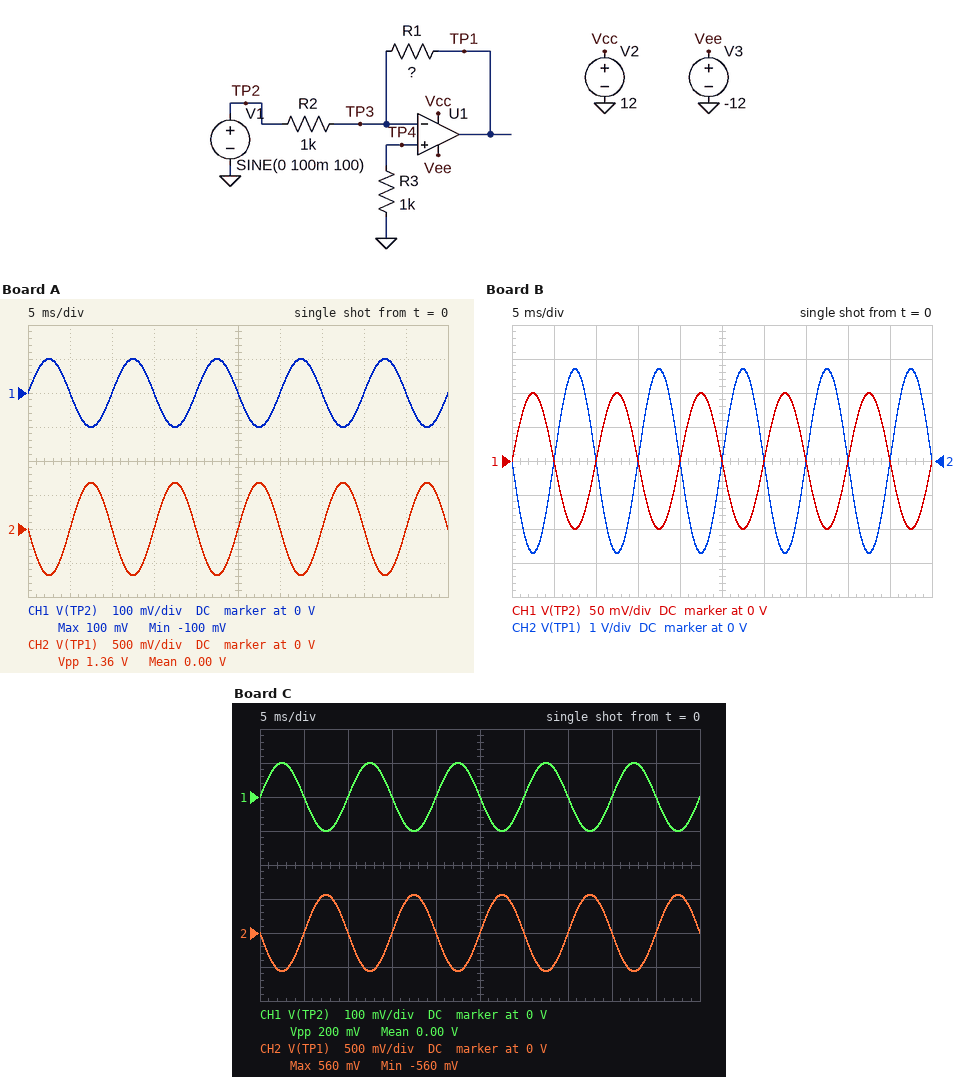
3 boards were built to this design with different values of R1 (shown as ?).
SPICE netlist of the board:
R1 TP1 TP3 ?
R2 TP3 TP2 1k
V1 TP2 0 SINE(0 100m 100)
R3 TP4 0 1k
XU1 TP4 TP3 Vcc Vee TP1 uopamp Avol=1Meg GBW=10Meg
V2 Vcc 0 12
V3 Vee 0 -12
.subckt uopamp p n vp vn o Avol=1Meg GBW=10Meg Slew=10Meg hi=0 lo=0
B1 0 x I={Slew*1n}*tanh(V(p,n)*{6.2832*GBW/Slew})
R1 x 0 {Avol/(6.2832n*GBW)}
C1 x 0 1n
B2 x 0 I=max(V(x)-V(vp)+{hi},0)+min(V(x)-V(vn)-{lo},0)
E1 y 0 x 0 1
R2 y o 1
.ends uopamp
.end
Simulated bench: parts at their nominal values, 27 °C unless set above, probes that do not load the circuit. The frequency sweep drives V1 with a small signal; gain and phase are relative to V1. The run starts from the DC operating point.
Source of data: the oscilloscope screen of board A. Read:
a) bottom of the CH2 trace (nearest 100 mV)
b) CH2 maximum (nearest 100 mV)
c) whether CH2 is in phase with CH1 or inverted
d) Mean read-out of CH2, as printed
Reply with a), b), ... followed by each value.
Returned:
a) -700 mV
b) 700 mV
c) inverted
d) 0.00 V
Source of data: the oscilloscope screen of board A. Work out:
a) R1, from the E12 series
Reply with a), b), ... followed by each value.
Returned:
a) 6.8 kΩ
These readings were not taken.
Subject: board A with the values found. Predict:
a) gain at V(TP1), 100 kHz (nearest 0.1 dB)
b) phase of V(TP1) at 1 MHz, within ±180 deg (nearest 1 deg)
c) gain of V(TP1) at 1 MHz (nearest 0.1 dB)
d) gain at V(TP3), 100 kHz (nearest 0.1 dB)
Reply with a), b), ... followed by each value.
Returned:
a) 16.6 dB
b) 142 deg
c) 14.6 dB
d) -23.4 dB
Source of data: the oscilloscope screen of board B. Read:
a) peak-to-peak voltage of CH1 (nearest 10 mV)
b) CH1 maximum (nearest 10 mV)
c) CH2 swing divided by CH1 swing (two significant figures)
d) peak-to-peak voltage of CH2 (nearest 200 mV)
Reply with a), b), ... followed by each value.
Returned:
a) 200 mV
b) 100 mV
c) 27
d) 5.4 V
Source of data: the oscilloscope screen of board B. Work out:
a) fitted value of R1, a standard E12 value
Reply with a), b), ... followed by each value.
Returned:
a) 27 kΩ
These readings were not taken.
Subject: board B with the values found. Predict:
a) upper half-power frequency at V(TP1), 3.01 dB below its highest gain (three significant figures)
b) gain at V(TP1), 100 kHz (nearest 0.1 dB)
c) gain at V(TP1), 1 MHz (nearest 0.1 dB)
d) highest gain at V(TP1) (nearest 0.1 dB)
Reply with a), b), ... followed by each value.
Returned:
a) 357 kHz
b) 28.3 dB
c) 19.2 dB
d) 28.6 dB
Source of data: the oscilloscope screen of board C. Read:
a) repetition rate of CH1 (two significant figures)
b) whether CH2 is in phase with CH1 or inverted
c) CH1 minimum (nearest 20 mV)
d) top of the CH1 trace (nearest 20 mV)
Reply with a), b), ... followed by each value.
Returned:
a) 100 Hz
b) inverted
c) -100 mV
d) 100 mV
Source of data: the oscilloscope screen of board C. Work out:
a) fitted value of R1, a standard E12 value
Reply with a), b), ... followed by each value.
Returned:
a) 5.6 kΩ
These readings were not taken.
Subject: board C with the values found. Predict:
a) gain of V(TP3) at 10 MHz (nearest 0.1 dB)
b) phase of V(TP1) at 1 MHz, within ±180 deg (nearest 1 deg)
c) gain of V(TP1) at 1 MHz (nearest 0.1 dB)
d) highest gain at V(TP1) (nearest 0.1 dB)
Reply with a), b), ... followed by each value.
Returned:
a) -1.5 dB
b) 147 deg
c) 13.4 dB
d) 15.0 dB
